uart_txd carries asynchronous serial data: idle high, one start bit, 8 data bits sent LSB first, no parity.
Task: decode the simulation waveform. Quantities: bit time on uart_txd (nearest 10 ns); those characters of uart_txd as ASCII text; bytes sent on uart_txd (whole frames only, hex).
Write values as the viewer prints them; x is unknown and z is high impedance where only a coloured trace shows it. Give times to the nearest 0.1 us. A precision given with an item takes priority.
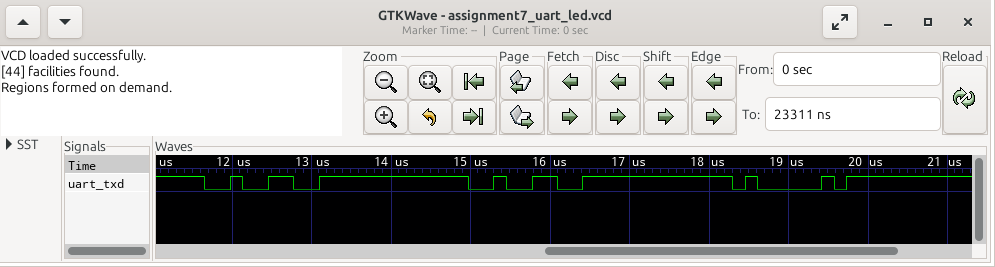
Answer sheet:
160 ns
"22A"
32, 32, 41
